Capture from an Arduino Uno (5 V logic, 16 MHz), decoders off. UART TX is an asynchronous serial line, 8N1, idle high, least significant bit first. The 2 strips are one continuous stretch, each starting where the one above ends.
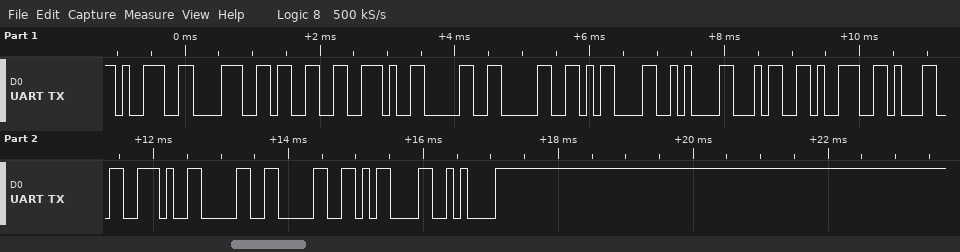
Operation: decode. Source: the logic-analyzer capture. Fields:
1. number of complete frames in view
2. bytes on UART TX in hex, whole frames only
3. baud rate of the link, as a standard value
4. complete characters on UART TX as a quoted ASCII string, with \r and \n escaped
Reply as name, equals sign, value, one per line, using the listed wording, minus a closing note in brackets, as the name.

number of complete frames in view = 16
bytes on UART TX in hex, whole frames only = 39 38 33 2E 30 30 0D 0A 34 39 31 2E 30 30 0D 0A
baud rate of the link, as a standard value = 9600 baud
complete characters on UART TX as a quoted ASCII string, with \r and \n escaped = "983.00\r\n491.00\r\n"
